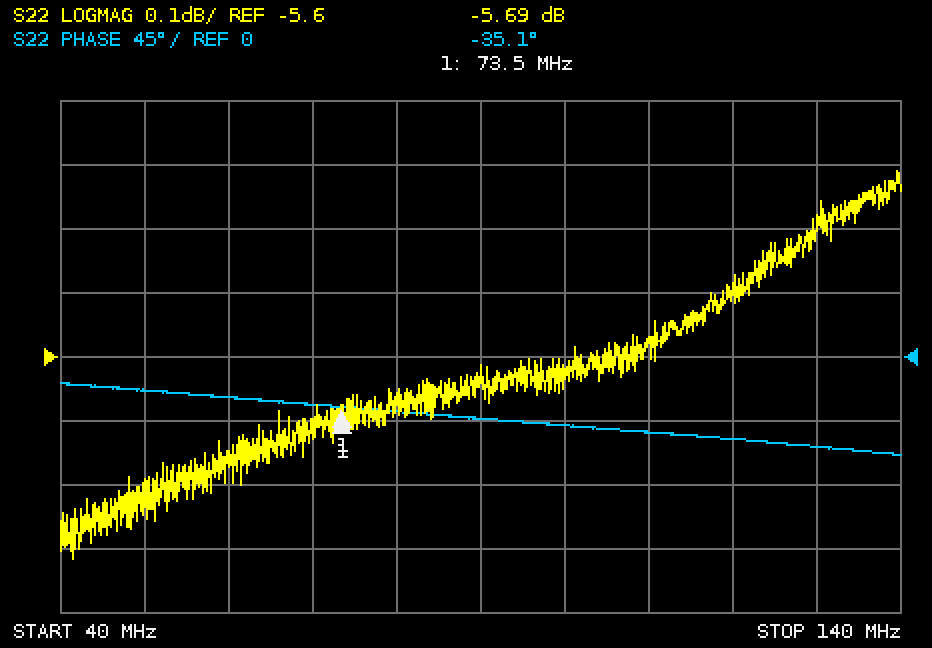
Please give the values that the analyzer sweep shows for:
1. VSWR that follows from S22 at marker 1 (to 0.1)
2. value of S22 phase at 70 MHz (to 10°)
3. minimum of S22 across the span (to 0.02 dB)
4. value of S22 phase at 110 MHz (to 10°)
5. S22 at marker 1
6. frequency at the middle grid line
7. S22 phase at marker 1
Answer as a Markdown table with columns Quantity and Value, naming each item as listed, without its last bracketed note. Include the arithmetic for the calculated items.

| Quantity | Value |
|---|---|
| VSWR that follows from S22 at marker 1 | (1 + 0.5194)/(1 − 0.5194) ≈ 3.2 |
| value of S22 phase at 70 MHz | -30° |
| minimum of S22 across the span | -5.92 dB |
| value of S22 phase at 110 MHz | -50° |
| S22 at marker 1 | -5.69 dB |
| frequency at the middle grid line | 90 MHz |
| S22 phase at marker 1 | -35.1° |
